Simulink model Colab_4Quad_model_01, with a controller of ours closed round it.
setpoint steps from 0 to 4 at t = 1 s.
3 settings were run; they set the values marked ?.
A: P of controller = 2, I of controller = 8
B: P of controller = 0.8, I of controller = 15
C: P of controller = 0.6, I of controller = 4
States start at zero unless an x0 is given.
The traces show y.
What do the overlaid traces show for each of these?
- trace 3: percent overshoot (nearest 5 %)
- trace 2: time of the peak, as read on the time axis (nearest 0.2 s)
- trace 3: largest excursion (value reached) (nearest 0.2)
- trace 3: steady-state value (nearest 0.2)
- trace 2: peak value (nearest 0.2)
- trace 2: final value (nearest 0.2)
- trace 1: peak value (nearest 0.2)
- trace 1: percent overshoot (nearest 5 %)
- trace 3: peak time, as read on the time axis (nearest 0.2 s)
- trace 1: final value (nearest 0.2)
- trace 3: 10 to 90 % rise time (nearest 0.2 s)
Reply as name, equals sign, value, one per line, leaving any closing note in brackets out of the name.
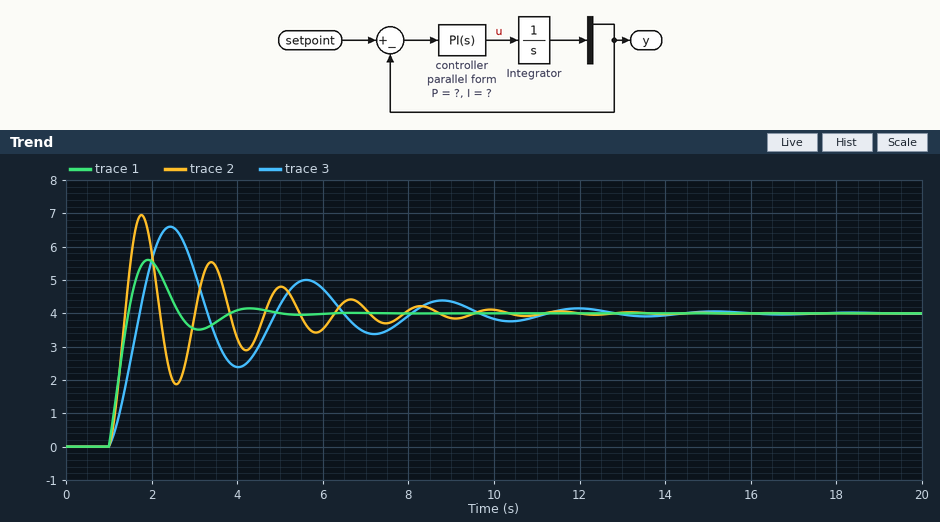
trace 3: percent overshoot = 65 %
trace 2: time of the peak, as read on the time axis = 1.8 s
trace 3: largest excursion (value reached) = 6.6
trace 3: steady-state value = 4.0
trace 2: peak value = 7.0
trace 2: final value = 4.0
trace 1: peak value = 5.6
trace 1: percent overshoot = 40 %
trace 3: peak time, as read on the time axis = 2.4 s
trace 1: final value = 4.0
trace 3: 10 to 90 % rise time = 0.6 s
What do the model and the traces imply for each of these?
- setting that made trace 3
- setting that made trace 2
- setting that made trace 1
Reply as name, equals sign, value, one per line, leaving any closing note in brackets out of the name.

setting that made trace 3 = C
setting that made trace 2 = B
setting that made trace 1 = A
